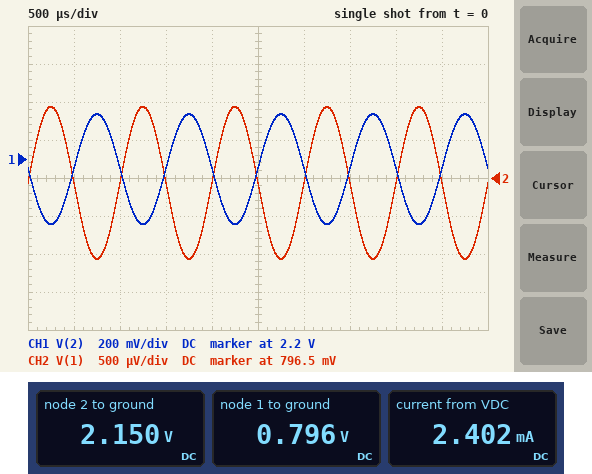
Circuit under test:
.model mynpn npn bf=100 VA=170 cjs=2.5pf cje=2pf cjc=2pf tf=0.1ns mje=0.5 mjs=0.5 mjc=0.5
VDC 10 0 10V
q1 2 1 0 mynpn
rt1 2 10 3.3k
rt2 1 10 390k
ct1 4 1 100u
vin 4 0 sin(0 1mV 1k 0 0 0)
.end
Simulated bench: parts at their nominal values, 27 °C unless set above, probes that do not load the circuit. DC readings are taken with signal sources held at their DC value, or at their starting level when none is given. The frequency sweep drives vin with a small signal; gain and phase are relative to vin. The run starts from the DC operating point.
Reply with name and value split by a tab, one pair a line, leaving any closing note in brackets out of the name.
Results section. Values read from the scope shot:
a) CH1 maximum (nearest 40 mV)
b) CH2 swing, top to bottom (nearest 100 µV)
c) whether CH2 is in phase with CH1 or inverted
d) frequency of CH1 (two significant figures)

CH1 maximum	2.44 V
CH2 swing, top to bottom	2.0 mV
whether CH2 is in phase with CH1 or inverted	inverted
frequency of CH1	1.0 kHz
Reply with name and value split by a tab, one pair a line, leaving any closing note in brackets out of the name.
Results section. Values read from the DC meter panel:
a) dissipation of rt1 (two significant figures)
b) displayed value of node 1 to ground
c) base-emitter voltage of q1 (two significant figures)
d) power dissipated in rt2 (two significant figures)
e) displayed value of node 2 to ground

dissipation of rt1	19 mW
displayed value of node 1 to ground	0.796 V
base-emitter voltage of q1	800 mV
power dissipated in rt2	220 µW
displayed value of node 2 to ground	2.150 V
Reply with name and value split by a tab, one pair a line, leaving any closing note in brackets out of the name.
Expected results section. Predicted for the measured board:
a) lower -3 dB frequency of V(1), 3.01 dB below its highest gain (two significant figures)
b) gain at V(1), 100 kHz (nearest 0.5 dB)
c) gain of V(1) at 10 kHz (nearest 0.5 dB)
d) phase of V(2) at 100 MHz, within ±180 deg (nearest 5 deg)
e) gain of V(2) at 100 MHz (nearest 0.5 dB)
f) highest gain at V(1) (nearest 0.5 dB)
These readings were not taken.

lower -3 dB frequency of V(1), 3.01 dB below its highest gain	1.5 Hz
gain at V(1), 100 kHz	0 dB
gain of V(1) at 10 kHz	0 dB
phase of V(2) at 100 MHz, within ±180 deg	100 deg
gain of V(2) at 100 MHz	35.5 dB
highest gain at V(1)	0 dB
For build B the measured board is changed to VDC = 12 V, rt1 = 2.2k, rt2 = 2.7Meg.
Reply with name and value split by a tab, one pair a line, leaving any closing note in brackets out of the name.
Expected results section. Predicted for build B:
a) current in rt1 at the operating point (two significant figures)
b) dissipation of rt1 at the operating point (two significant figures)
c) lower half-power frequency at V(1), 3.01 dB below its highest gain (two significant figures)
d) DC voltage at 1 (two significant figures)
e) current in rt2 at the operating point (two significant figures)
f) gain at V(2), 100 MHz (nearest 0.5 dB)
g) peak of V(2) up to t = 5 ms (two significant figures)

current in rt1 at the operating point	440 µA
dissipation of rt1 at the operating point	430 µW
lower half-power frequency at V(1), 3.01 dB below its highest gain	260 mHz
DC voltage at 1	750 mV
current in rt2 at the operating point	4.2 µA
gain at V(2), 100 MHz	26.0 dB
peak of V(2) up to t = 5 ms	11 V
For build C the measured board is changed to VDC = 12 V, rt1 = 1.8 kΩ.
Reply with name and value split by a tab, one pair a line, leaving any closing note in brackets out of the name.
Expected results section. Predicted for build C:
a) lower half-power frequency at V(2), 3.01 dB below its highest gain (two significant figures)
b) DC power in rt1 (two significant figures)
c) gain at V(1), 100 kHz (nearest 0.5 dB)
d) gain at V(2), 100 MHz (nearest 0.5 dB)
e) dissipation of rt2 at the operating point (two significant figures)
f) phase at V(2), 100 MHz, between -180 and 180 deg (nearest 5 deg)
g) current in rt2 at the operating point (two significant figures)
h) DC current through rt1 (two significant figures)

lower half-power frequency at V(2), 3.01 dB below its highest gain	1.8 Hz
DC power in rt1	16 mW
gain at V(1), 100 kHz	0 dB
gain at V(2), 100 MHz	40.5 dB
dissipation of rt2 at the operating point	320 µW
phase at V(2), 100 MHz, between -180 and 180 deg	120 deg
current in rt2 at the operating point	29 µA
DC current through rt1	3.0 mA
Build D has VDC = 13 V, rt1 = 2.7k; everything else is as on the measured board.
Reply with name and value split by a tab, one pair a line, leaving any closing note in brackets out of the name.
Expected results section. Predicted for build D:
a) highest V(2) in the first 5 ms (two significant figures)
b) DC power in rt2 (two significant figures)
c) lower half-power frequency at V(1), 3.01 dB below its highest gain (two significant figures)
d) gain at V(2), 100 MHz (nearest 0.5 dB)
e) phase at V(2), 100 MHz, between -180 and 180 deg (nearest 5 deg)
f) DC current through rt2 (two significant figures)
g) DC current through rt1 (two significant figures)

highest V(2) in the first 5 ms	4.7 V
DC power in rt2	380 µW
lower half-power frequency at V(1), 3.01 dB below its highest gain	1.9 Hz
gain at V(2), 100 MHz	40.5 dB
phase at V(2), 100 MHz, between -180 and 180 deg	110 deg
DC current through rt2	31 µA
DC current through rt1	3.2 mA
